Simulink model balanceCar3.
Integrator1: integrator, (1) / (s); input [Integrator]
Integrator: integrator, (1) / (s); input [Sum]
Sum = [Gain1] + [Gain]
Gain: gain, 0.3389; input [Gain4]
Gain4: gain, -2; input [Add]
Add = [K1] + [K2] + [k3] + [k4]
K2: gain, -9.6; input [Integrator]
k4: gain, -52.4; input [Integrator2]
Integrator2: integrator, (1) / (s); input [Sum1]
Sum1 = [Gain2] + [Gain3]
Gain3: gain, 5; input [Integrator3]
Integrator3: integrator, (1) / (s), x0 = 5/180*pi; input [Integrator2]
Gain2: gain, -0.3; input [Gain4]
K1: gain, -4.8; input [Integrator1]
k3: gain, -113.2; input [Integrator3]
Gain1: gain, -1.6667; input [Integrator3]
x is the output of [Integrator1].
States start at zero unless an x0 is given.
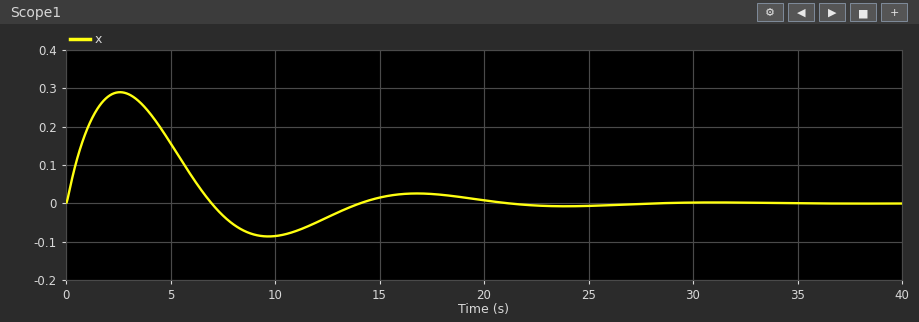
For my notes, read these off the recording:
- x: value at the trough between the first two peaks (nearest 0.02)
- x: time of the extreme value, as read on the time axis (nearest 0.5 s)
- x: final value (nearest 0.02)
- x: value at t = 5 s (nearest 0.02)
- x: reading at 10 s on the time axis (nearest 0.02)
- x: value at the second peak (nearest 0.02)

-0.08
2.5 s
0.00
0.16
-0.08
0.02
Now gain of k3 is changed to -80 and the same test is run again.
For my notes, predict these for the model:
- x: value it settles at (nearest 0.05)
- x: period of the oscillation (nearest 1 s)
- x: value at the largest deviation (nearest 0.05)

0.00
11 s
0.35
